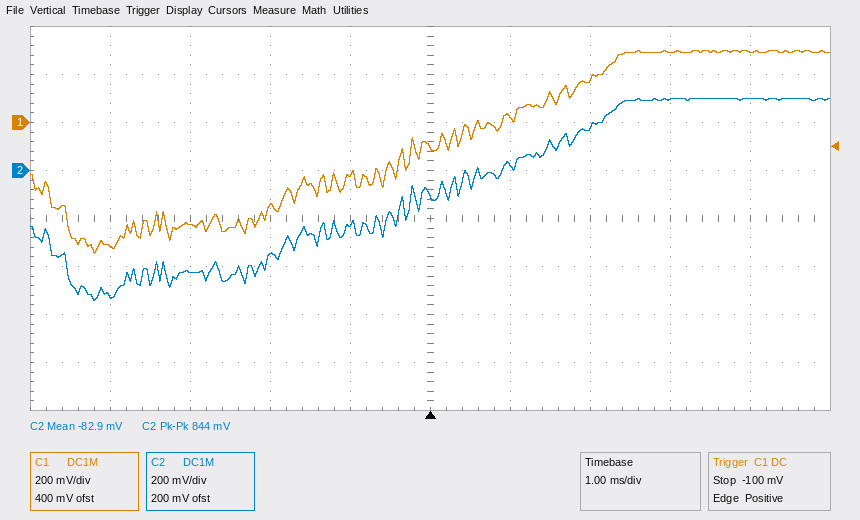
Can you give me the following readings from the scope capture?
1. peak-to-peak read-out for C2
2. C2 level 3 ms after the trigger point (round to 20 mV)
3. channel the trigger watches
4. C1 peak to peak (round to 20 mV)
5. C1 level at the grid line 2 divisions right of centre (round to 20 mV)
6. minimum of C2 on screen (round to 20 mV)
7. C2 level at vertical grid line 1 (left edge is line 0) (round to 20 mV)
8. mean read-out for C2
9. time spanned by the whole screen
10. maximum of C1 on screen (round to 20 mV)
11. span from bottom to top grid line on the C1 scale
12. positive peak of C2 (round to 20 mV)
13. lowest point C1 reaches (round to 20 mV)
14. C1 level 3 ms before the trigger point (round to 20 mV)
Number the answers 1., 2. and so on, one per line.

1. 844 mV
2. 300 mV
3. C1
4. 840 mV
5. 180 mV
6. -540 mV
7. -520 mV
8. -82.9 mV
9. 10 ms
10. 300 mV
11. 1.6 V
12. 300 mV
13. -540 mV
14. -420 mV
